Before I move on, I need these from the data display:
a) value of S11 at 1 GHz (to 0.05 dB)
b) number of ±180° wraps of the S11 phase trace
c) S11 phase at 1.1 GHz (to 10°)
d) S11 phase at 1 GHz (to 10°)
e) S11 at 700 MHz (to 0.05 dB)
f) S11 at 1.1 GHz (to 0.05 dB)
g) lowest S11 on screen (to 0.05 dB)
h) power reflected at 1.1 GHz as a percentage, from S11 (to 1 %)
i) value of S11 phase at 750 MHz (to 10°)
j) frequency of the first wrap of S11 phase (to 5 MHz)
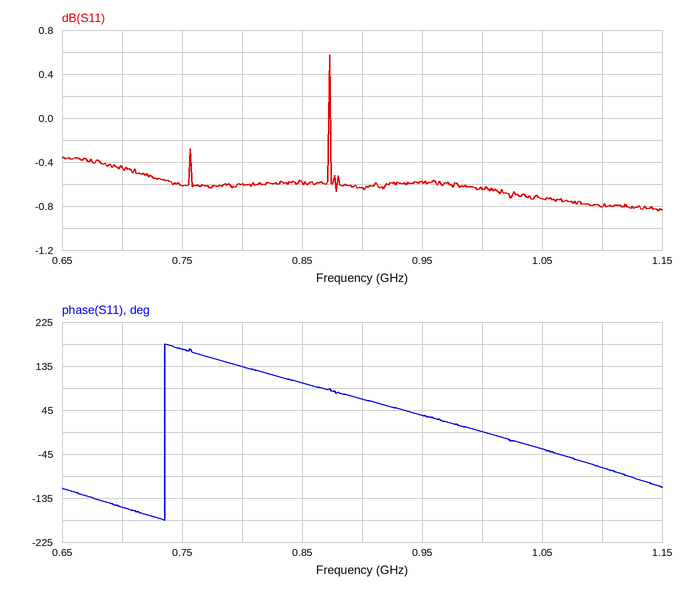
-0.65 dB
1
-70°
0°
-0.45 dB
-0.80 dB
-0.85 dB
83 %
170°
735 MHz
